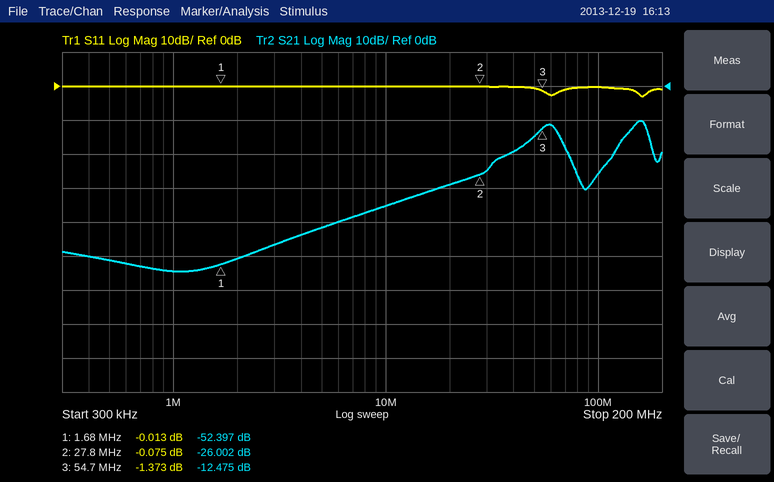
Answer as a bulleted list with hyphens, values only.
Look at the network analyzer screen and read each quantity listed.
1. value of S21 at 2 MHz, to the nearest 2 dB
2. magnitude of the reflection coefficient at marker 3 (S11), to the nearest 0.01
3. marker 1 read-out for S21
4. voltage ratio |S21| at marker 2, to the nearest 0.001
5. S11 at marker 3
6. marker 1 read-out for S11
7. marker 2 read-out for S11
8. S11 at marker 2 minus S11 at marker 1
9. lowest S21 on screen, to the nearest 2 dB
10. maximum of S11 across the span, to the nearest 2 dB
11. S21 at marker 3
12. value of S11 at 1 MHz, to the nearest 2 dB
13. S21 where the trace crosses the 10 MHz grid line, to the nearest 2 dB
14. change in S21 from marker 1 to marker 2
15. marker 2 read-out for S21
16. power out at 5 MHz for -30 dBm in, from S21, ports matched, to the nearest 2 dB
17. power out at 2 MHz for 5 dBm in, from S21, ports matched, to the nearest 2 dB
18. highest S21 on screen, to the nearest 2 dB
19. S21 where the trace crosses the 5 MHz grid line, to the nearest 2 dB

- -50 dB
- 0.85
- -52.397 dB
- 0.050
- -1.373 dB
- -0.013 dB
- -0.075 dB
- -0.062 dB
- -54 dB
- 0 dB
- -12.475 dB
- 0 dB
- -36 dB
- 26.395 dB
- -26.002 dB
- -72 dBm
- -46 dBm
- -10 dB
- -42 dB
